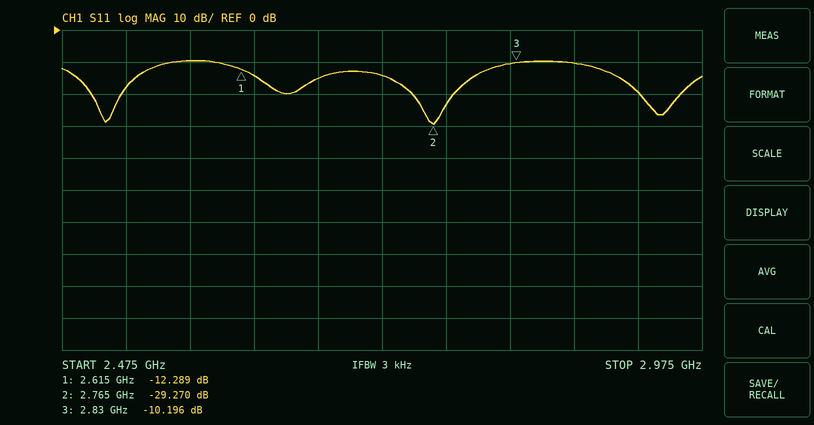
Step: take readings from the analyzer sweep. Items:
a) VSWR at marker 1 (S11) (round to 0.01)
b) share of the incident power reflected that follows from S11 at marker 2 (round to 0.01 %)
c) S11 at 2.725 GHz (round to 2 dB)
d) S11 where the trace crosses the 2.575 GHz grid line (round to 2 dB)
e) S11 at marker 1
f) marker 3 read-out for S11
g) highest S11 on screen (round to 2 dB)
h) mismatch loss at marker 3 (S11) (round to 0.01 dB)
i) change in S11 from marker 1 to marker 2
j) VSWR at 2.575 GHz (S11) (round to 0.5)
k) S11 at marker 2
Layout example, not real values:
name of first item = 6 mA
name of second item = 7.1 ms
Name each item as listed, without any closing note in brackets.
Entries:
VSWR at marker 1 (S11) = 1.64
share of the incident power reflected that follows from S11 at marker 2 = 0.12 %
S11 at 2.725 GHz = -14 dB
S11 where the trace crosses the 2.575 GHz grid line = -10 dB
S11 at marker 1 = -12.289 dB
marker 3 read-out for S11 = -10.196 dB
highest S11 on screen = -10 dB
mismatch loss at marker 3 (S11) = 0.44 dB
change in S11 from marker 1 to marker 2 = -16.981 dB
VSWR at 2.575 GHz (S11) = 2.0
S11 at marker 2 = -29.270 dB
